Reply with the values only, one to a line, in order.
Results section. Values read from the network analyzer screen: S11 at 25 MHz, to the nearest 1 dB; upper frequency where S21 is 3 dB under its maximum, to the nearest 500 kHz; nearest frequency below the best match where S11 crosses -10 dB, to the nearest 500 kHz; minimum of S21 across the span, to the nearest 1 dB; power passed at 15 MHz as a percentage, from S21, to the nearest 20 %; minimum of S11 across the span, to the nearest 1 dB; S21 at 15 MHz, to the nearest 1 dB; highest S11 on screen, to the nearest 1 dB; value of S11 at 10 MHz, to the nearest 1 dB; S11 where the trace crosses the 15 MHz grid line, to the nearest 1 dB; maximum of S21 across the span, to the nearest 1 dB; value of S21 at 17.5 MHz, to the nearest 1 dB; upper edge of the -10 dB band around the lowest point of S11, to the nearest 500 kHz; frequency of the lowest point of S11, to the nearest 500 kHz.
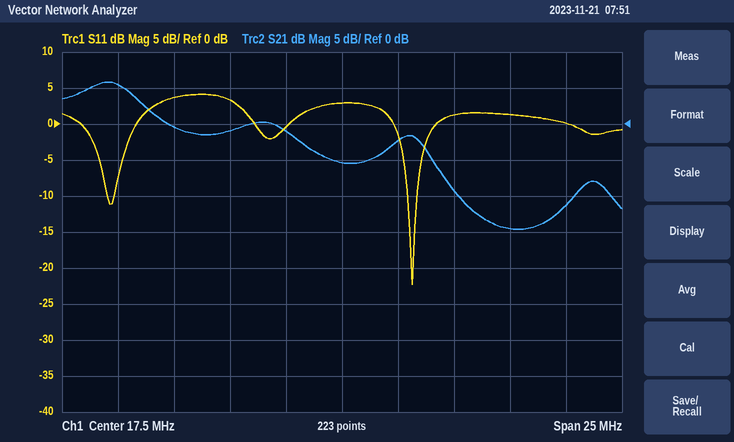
1 dB
8.5 MHz
20.5 MHz
-15 dB
80 %
-22 dB
-1 dB
4 dB
4 dB
0 dB
6 dB
-5 dB
21.0 MHz
20.5 MHz
